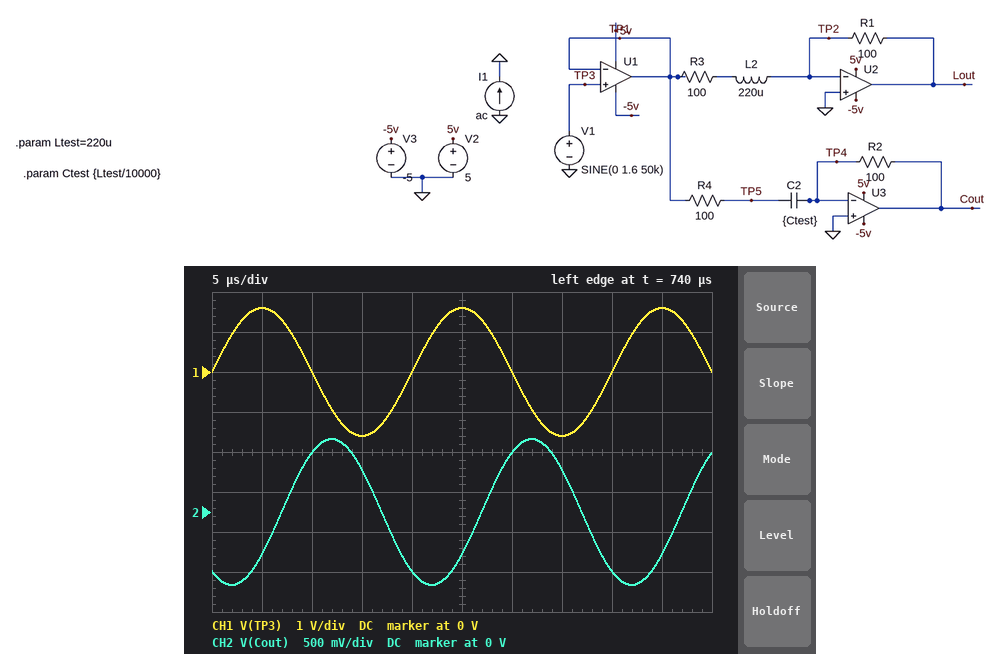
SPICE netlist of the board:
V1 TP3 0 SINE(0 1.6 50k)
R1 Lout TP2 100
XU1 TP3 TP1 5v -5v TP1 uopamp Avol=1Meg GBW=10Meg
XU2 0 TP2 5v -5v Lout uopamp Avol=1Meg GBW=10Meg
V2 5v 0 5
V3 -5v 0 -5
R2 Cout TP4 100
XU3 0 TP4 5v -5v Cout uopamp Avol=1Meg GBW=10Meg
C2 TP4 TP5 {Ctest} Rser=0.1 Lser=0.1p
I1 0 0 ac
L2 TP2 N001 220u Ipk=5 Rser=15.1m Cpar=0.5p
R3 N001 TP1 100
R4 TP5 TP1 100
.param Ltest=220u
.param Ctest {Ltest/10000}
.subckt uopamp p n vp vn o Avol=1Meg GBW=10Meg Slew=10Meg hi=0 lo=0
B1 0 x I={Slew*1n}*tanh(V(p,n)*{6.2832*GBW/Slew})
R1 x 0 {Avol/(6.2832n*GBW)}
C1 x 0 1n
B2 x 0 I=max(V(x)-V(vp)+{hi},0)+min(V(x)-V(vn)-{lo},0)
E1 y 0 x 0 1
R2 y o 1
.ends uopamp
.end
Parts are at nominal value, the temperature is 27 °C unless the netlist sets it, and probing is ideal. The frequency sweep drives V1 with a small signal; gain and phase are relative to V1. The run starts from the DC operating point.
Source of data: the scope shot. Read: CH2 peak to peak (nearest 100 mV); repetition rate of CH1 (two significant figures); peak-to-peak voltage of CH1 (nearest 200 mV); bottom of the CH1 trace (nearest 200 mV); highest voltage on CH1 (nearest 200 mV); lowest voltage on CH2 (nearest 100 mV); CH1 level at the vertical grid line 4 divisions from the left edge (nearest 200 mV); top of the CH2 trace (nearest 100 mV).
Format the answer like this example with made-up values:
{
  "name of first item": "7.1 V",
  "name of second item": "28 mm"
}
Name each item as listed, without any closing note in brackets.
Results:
{
  "CH2 peak to peak": "1.8 V",
  "repetition rate of CH1": "50 kHz",
  "peak-to-peak voltage of CH1": "3.2 V",
  "bottom of the CH1 trace": "-1.6 V",
  "highest voltage on CH1": "1.6 V",
  "lowest voltage on CH2": "-900 mV",
  "CH1 level at the vertical grid line 4 divisions from the left edge": "0 V",
  "top of the CH2 trace": "900 mV"
}
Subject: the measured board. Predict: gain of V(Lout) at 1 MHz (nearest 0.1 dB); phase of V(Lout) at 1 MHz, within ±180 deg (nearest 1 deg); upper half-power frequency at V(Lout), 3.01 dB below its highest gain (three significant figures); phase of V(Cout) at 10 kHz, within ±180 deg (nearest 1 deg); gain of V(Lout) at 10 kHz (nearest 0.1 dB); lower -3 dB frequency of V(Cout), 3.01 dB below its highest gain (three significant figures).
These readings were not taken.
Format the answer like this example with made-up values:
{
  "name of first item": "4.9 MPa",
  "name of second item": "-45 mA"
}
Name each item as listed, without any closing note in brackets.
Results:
{
  "gain of V(Lout) at 1 MHz": "-23.0 dB",
  "phase of V(Lout) at 1 MHz, within ±180 deg": "83 deg",
  "upper half-power frequency at V(Lout), 3.01 dB below its highest gain": "71.8 kHz",
  "phase of V(Cout) at 10 kHz, within ±180 deg": "-98 deg",
  "gain of V(Lout) at 10 kHz": "-0.1 dB",
  "lower -3 dB frequency of V(Cout), 3.01 dB below its highest gain": "70.5 kHz"
}
